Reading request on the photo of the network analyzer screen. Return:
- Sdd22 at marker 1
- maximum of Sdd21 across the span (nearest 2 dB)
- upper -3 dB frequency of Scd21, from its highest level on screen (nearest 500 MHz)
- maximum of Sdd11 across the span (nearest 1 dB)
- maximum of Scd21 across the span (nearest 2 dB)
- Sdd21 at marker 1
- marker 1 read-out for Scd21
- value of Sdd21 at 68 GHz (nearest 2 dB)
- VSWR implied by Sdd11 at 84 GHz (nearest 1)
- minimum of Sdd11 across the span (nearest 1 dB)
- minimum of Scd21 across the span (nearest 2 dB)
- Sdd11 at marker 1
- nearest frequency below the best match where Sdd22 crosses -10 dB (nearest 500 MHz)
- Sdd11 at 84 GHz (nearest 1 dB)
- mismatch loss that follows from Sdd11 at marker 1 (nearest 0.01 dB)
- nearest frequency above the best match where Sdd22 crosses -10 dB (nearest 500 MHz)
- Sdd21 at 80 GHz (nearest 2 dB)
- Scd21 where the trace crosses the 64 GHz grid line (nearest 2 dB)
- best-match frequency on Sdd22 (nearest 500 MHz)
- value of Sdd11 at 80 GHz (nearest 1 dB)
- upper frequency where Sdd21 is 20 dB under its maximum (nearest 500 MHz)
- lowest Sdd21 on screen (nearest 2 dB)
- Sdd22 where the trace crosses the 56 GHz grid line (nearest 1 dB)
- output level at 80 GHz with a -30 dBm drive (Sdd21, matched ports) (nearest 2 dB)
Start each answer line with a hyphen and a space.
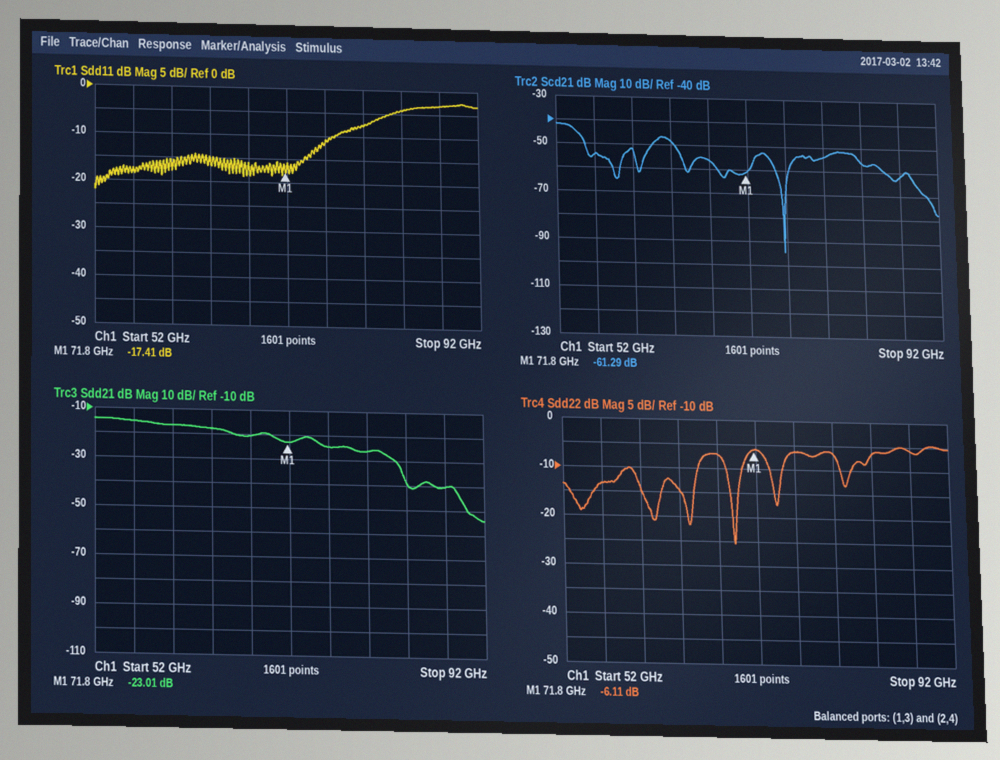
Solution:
- -6.11 dB
- -14 dB
- 54.0 GHz
- -3 dB
- -42 dB
- -23.01 dB
- -61.29 dB
- -20 dB
- 4
- -22 dB
- -94 dB
- -17.41 dB
- 69.0 GHz
- -4 dB
- 0.08 dB
- 70.5 GHz
- -26 dB
- -48 dB
- 69.5 GHz
- -8 dB
- 83.5 GHz
- -54 dB
- -13 dB
- -56 dBm
